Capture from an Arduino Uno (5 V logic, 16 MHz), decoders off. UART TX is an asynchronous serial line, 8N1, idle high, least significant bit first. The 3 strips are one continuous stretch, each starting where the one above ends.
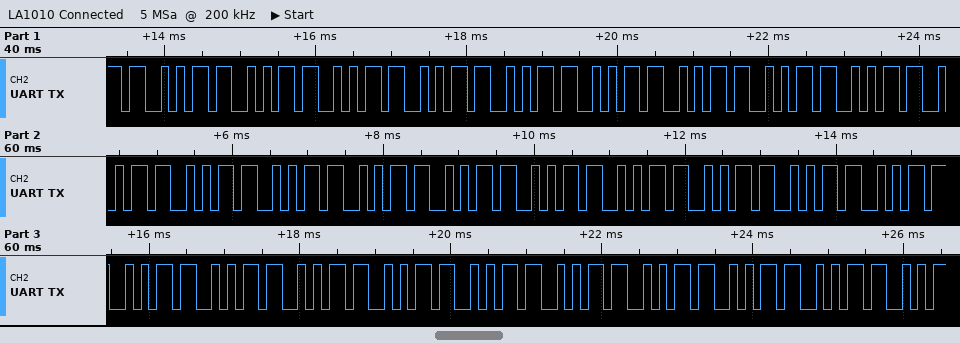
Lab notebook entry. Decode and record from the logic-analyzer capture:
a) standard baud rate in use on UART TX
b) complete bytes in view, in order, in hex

9600 baud
0x53 0x53 0x53 0x53 0x53 0x53 0x53 0x53 0x53 0x53 0x53 0x53 0x53 0x53 0x53 0x53 0x53 0x53 0x53 0x53 0x53 0x53 0x53 0x53 0x53 0x53 0x53 0x53 0x53
